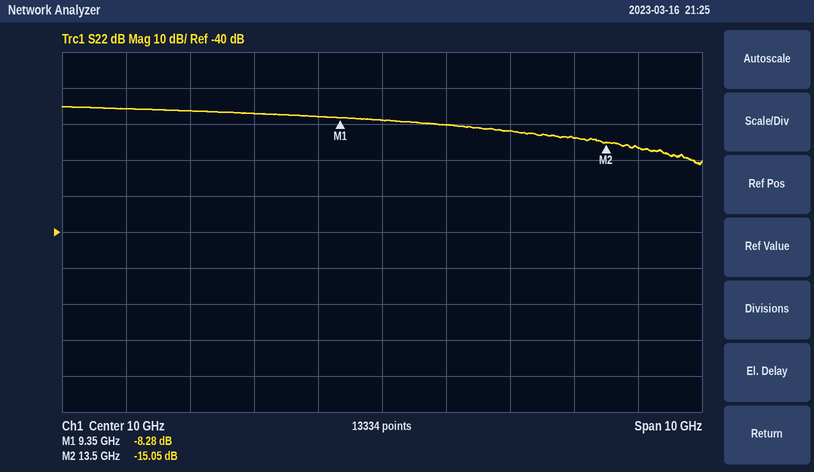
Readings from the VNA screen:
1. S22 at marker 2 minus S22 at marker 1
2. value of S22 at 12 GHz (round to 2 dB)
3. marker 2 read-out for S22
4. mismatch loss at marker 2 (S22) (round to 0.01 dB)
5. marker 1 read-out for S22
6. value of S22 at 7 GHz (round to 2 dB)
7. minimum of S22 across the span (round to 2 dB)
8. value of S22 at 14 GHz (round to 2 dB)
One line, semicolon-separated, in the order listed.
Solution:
-6.77 dB; -12 dB; -15.05 dB; 0.14 dB; -8.28 dB; -6 dB; -22 dB; -16 dB
